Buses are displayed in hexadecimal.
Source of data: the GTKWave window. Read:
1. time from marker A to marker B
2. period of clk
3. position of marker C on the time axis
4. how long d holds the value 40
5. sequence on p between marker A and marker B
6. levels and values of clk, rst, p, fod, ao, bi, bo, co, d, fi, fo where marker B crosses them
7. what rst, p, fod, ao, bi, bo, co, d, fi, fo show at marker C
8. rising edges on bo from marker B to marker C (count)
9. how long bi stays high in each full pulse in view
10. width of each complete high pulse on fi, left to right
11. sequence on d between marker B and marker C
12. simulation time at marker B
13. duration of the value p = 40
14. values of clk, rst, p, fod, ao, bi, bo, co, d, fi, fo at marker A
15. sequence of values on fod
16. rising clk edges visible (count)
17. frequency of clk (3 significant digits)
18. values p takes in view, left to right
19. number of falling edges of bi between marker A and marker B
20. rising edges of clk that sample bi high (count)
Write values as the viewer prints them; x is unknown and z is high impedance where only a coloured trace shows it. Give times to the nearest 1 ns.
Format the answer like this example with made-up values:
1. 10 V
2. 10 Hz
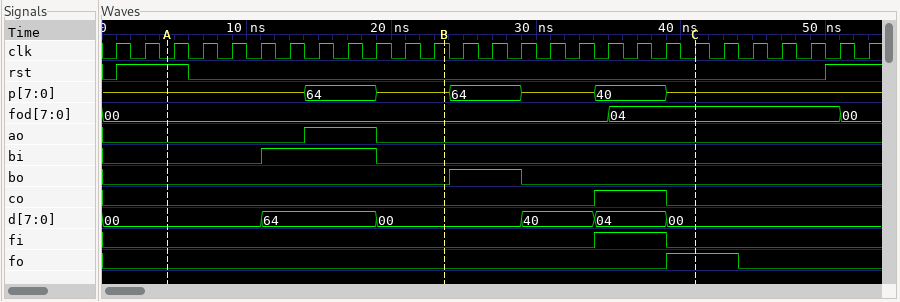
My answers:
1. 19 ns
2. 2 ns
3. 41 ns
4. 5 ns
5. z, 64, z
6. clk=1, rst=0, p=z, fod=00, ao=0, bi=0, bo=0, co=0, d=00, fi=0, fo=0
7. rst=0, p=z, fod=04, ao=0, bi=0, bo=0, co=0, d=00, fi=0, fo=1
8. 1
9. 8 ns
10. 5 ns
11. 00, 40, 04, 00
12. 24 ns
13. 5 ns
14. clk=0, rst=1, p=z, fod=00, ao=0, bi=0, bo=0, co=0, d=00, fi=0, fo=0
15. 00, 04, 00
16. 27
17. 500 MHz
18. z, 64, z, 64, z, 40, z
19. 1
20. 4
